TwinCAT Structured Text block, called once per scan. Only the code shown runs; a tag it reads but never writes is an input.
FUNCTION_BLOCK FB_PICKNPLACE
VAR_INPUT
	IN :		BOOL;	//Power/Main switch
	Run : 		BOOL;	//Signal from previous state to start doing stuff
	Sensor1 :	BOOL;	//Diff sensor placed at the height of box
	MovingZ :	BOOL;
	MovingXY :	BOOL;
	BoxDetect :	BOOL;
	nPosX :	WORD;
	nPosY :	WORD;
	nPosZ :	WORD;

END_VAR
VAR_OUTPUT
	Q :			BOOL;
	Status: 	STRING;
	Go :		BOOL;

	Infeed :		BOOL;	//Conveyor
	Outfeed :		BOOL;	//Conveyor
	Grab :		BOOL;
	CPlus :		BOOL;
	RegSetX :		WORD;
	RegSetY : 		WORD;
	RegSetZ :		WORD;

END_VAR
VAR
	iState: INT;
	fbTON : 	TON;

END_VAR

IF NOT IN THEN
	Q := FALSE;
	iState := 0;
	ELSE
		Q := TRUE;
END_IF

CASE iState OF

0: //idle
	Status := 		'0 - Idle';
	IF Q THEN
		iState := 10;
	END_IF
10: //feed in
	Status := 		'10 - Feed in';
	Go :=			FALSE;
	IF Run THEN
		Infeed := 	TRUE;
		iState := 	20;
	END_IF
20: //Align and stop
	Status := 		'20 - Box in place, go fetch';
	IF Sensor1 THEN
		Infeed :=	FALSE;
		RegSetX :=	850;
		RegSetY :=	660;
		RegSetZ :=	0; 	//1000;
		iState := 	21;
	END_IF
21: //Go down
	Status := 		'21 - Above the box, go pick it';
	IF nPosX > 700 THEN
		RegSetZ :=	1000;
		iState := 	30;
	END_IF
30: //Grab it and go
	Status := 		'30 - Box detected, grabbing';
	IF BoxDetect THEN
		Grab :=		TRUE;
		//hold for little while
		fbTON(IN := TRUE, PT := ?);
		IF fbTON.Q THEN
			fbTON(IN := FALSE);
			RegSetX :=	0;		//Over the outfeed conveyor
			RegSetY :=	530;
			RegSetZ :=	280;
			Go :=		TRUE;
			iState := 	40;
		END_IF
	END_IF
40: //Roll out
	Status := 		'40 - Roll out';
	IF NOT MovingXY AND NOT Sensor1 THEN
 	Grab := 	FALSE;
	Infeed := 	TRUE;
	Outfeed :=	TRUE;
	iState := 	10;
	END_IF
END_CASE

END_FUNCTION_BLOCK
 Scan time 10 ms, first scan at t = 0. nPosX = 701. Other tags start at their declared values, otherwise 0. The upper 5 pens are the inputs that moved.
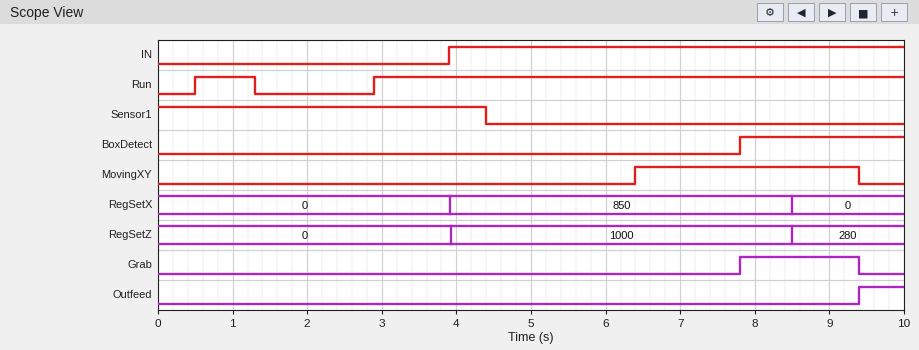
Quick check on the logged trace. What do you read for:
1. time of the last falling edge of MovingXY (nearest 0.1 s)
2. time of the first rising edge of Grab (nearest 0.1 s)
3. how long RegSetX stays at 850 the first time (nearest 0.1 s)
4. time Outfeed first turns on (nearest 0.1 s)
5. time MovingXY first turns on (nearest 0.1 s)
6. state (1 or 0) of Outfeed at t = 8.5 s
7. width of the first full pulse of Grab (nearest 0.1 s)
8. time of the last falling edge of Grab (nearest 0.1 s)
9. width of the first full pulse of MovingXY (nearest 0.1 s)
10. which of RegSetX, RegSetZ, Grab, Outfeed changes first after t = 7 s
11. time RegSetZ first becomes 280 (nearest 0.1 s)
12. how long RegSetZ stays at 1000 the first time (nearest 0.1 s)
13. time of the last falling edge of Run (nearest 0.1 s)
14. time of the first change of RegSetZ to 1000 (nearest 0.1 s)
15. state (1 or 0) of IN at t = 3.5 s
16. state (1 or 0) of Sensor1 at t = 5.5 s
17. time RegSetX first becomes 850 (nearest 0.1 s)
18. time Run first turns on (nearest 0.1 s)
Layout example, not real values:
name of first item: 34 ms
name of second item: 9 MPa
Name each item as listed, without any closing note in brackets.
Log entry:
time of the last falling edge of MovingXY: 9.4 s
time of the first rising edge of Grab: 7.8 s
how long RegSetX stays at 850 the first time: 4.6 s
time Outfeed first turns on: 9.4 s
time MovingXY first turns on: 6.4 s
state (1 or 0) of Outfeed at t = 8.5 s: 0
width of the first full pulse of Grab: 1.6 s
time of the last falling edge of Grab: 9.4 s
width of the first full pulse of MovingXY: 3.0 s
which of RegSetX, RegSetZ, Grab, Outfeed changes first after t = 7 s: Grab
time RegSetZ first becomes 280: 8.5 s
how long RegSetZ stays at 1000 the first time: 4.6 s
time of the last falling edge of Run: 1.3 s
time of the first change of RegSetZ to 1000: 3.9 s
state (1 or 0) of IN at t = 3.5 s: 0
state (1 or 0) of Sensor1 at t = 5.5 s: 0
time RegSetX first becomes 850: 3.9 s
time Run first turns on: 0.5 s
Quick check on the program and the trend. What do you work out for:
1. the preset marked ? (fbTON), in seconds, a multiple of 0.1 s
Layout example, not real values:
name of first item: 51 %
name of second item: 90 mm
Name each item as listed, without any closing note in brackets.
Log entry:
the preset marked ? (fbTON), in seconds, a multiple of 0.1 s: 0.7 s
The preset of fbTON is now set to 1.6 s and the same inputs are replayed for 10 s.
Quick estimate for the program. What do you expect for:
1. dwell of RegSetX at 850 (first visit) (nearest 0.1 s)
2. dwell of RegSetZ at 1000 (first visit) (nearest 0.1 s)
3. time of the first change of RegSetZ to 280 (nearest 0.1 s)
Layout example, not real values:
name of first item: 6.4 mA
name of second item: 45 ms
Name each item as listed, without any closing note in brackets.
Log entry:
dwell of RegSetX at 850 (first visit): 5.5 s
dwell of RegSetZ at 1000 (first visit): 5.5 s
time of the first change of RegSetZ to 280: 9.4 s
